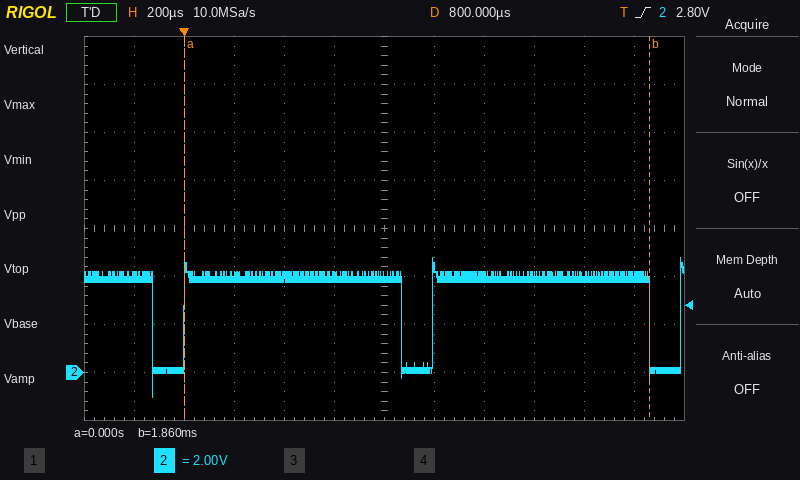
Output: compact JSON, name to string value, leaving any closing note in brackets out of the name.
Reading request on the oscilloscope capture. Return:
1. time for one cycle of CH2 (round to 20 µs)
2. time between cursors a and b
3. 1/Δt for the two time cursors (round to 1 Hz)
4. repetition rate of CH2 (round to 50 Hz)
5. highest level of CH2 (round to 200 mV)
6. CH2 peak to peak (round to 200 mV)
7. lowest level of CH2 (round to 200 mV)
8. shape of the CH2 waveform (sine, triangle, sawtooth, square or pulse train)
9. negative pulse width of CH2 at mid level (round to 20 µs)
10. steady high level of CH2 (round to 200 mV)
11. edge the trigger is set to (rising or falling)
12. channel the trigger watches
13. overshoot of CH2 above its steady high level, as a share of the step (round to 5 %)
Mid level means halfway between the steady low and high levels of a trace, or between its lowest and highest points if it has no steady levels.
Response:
{"time for one cycle of CH2": "1.00 ms", "time between cursors a and b": "1.86 ms", "1/Δt for the two time cursors": "538 Hz", "repetition rate of CH2": "1.00 kHz", "highest level of CH2": "4.8 V", "CH2 peak to peak": "5.8 V", "lowest level of CH2": "-1.0 V", "shape of the CH2 waveform": "pulse train", "negative pulse width of CH2 at mid level": "120 µs", "steady high level of CH2": "4.0 V", "edge the trigger is set to": "rising", "channel the trigger watches": "CH2", "overshoot of CH2 above its steady high level, as a share of the step": "20 %"}
